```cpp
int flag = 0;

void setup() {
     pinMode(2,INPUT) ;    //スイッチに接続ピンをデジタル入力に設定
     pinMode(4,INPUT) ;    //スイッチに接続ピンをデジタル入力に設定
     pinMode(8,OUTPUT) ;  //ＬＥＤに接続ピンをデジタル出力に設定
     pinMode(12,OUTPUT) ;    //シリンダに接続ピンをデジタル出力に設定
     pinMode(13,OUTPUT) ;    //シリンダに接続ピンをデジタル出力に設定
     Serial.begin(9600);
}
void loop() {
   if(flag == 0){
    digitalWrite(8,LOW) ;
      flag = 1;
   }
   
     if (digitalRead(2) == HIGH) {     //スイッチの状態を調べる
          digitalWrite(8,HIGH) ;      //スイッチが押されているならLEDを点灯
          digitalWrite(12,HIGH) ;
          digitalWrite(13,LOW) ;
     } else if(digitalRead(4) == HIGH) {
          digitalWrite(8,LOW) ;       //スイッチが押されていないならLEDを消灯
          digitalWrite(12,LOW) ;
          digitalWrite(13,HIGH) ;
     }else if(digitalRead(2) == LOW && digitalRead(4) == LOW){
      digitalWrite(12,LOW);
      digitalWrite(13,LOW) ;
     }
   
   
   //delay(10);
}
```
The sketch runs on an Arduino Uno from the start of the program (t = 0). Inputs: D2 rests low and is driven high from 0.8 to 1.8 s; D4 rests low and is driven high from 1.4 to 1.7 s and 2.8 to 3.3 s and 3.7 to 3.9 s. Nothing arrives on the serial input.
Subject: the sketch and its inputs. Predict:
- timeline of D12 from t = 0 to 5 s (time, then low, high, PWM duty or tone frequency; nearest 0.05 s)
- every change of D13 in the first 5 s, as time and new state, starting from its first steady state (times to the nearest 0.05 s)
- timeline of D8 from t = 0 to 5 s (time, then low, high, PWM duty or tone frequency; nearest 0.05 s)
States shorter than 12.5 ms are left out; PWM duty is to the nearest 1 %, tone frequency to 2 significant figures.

0 s low; 0.8 s high; 1.8 s low
0 s low; 2.8 s high; 3.3 s low; 3.7 s high; 3.9 s low
0 s low; 0.8 s high; 2.8 s low
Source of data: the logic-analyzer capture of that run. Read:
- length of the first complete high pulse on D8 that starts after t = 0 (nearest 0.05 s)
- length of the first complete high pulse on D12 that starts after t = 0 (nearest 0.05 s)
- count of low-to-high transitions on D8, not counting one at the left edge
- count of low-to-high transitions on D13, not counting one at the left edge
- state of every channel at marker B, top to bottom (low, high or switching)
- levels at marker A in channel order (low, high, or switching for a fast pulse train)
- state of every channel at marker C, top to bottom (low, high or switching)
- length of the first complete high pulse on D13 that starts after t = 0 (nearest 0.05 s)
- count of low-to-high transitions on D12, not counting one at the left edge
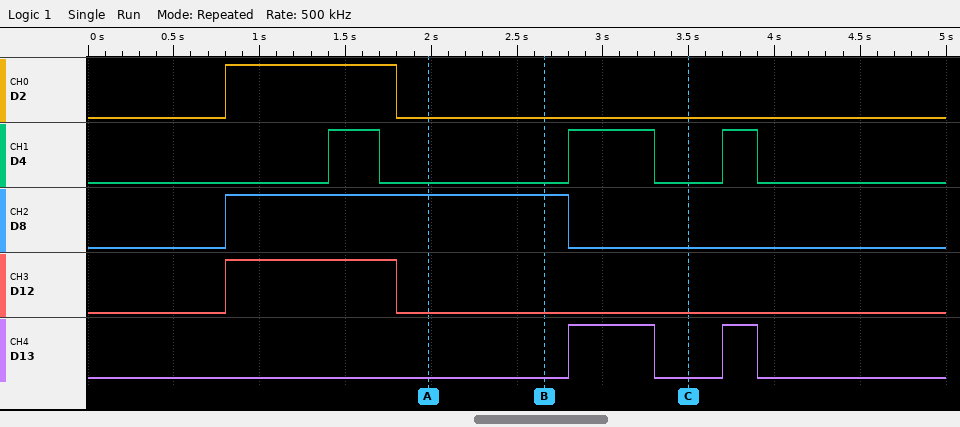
2.00 s
1.00 s
1
2
D2 low, D4 low, D8 high, D12 low, D13 low
D2 low, D4 low, D8 high, D12 low, D13 low
D2 low, D4 low, D8 low, D12 low, D13 low
0.50 s
1
